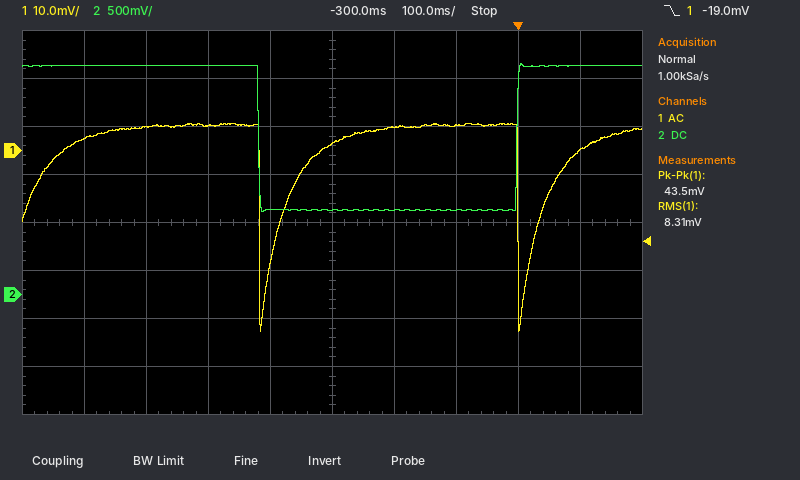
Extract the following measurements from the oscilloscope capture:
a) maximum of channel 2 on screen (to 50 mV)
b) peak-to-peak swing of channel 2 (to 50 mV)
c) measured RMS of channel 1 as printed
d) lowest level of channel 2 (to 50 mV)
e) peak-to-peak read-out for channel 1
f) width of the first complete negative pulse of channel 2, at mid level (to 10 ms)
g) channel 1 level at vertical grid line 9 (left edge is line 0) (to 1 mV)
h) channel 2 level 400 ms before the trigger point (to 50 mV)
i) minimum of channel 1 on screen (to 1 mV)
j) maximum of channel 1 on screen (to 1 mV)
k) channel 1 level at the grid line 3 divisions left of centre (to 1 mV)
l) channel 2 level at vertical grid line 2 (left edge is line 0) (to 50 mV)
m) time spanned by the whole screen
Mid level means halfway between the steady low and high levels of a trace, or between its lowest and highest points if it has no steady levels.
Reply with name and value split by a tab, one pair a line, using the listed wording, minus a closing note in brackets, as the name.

maximum of channel 2 on screen	2.40 V
peak-to-peak swing of channel 2	1.55 V
measured RMS of channel 1 as printed	8.31 mV
lowest level of channel 2	850 mV
peak-to-peak read-out for channel 1	43.5 mV
width of the first complete negative pulse of channel 2, at mid level	420 ms
channel 1 level at vertical grid line 9 (left edge is line 0)	0 mV
channel 2 level 400 ms before the trigger point	900 mV
minimum of channel 1 on screen	-38 mV
maximum of channel 1 on screen	6 mV
channel 1 level at the grid line 3 divisions left of centre	5 mV
channel 2 level at vertical grid line 2 (left edge is line 0)	2.40 V
time spanned by the whole screen	1 s
